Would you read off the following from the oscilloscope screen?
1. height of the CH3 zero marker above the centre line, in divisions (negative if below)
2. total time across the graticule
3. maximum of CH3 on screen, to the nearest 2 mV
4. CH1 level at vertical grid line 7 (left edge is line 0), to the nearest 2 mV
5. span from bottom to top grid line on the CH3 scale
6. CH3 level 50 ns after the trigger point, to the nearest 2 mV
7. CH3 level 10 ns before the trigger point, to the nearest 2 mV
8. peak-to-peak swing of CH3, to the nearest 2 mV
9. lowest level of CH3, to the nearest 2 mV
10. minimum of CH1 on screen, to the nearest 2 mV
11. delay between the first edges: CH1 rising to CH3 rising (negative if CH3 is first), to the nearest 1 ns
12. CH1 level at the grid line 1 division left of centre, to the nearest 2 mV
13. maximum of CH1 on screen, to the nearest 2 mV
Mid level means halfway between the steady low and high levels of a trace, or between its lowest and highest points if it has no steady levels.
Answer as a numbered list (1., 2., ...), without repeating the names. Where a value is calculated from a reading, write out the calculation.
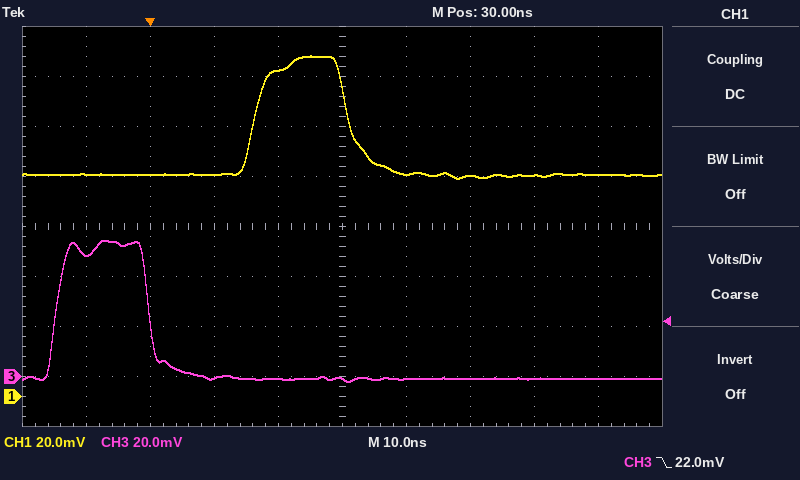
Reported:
1. -3.0 div
2. 100 ns
3. 54 mV
4. 88 mV
5. 160 mV
6. 0 mV
7. 48 mV
8. 54 mV − (-2 mV) = 56 mV
9. -2 mV
10. 88 mV
11. -31 ns
12. 130 mV
13. 136 mV
